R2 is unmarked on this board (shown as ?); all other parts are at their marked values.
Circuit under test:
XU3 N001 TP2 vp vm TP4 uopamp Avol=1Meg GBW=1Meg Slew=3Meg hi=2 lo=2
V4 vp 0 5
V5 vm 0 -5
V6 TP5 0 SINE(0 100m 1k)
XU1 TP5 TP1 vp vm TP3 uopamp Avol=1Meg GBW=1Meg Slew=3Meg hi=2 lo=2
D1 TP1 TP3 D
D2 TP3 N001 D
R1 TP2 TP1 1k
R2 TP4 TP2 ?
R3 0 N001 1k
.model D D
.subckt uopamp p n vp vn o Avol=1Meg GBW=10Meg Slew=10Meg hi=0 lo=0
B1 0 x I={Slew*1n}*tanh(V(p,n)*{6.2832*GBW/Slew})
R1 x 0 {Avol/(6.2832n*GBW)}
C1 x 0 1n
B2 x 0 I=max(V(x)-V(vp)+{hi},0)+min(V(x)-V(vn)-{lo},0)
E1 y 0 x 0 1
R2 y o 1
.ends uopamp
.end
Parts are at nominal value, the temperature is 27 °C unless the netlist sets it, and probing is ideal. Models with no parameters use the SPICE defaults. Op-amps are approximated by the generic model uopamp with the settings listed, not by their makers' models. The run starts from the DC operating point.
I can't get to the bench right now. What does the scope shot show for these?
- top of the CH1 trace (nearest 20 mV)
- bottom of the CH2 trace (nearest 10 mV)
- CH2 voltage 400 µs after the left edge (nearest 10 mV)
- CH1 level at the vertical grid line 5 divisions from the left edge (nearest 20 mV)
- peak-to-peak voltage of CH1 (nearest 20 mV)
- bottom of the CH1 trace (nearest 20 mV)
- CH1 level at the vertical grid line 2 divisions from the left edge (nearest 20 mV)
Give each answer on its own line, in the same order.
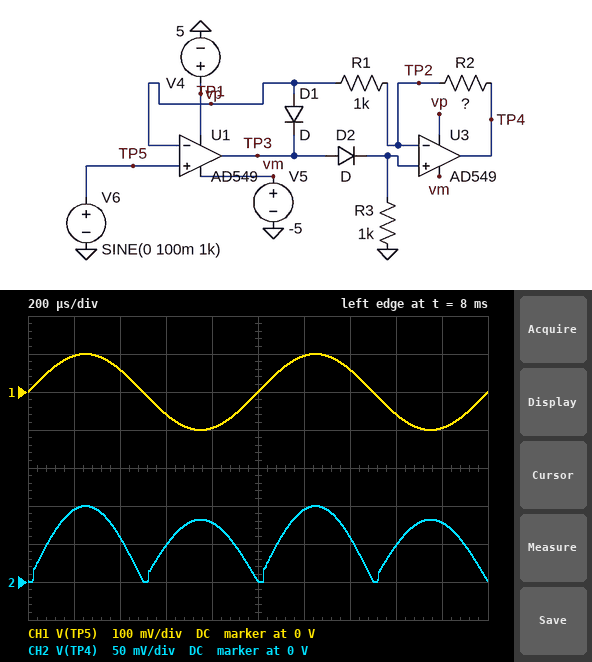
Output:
100 mV
0 V
60 mV
0 V
200 mV
-100 mV
60 mV
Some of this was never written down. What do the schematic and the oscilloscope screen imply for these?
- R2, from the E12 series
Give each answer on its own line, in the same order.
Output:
820 Ω
